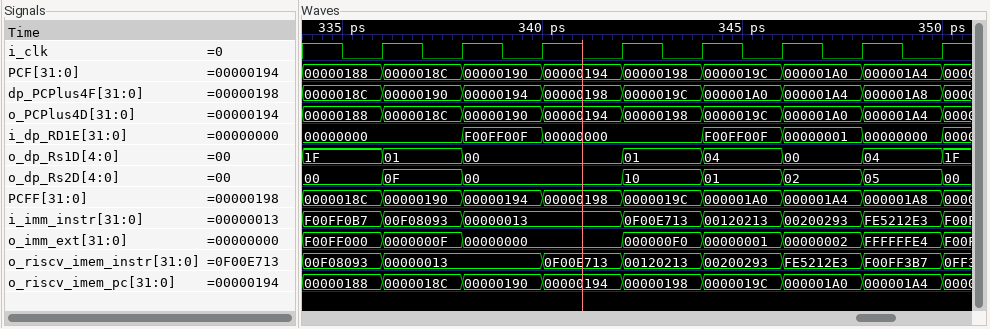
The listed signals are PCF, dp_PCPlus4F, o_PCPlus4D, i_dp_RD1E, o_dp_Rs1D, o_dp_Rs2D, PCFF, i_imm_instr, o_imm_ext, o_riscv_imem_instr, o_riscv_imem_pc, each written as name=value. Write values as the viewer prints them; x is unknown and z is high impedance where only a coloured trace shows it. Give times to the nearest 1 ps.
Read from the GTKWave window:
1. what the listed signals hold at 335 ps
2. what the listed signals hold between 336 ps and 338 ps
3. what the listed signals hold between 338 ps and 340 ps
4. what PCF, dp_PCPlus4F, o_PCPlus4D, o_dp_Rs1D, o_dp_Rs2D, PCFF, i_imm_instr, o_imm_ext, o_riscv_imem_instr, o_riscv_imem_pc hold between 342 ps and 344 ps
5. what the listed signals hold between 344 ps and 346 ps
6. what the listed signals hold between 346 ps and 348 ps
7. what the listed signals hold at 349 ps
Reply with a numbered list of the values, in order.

1. PCF=00000188, dp_PCPlus4F=0000018C, o_PCPlus4D=00000188, i_dp_RD1E=00000000, o_dp_Rs1D=1F, o_dp_Rs2D=00, PCFF=0000018C, i_imm_instr=F00FF0B7, o_imm_ext=F00FF000, o_riscv_imem_instr=00F08093, o_riscv_imem_pc=00000188
2. PCF=0000018C, dp_PCPlus4F=00000190, o_PCPlus4D=0000018C, i_dp_RD1E=00000000, o_dp_Rs1D=01, o_dp_Rs2D=0F, PCFF=00000190, i_imm_instr=00F08093, o_imm_ext=0000000F, o_riscv_imem_instr=00000013, o_riscv_imem_pc=0000018C
3. PCF=00000190, dp_PCPlus4F=00000194, o_PCPlus4D=00000190, i_dp_RD1E=F00FF00F, o_dp_Rs1D=00, o_dp_Rs2D=00, PCFF=00000194, i_imm_instr=00000013, o_imm_ext=00000000, o_riscv_imem_instr=00000013, o_riscv_imem_pc=00000190
4. PCF=00000198, dp_PCPlus4F=0000019C, o_PCPlus4D=00000198, o_dp_Rs1D=01, o_dp_Rs2D=10, PCFF=0000019C, i_imm_instr=0F00E713, o_imm_ext=000000F0, o_riscv_imem_instr=00120213, o_riscv_imem_pc=00000198
5. PCF=0000019C, dp_PCPlus4F=000001A0, o_PCPlus4D=0000019C, i_dp_RD1E=F00FF00F, o_dp_Rs1D=04, o_dp_Rs2D=01, PCFF=000001A0, i_imm_instr=00120213, o_imm_ext=00000001, o_riscv_imem_instr=00200293, o_riscv_imem_pc=0000019C
6. PCF=000001A0, dp_PCPlus4F=000001A4, o_PCPlus4D=000001A0, i_dp_RD1E=00000001, o_dp_Rs1D=00, o_dp_Rs2D=02, PCFF=000001A4, i_imm_instr=00200293, o_imm_ext=00000002, o_riscv_imem_instr=FE5212E3, o_riscv_imem_pc=000001A0
7. PCF=000001A4, dp_PCPlus4F=000001A8, o_PCPlus4D=000001A4, i_dp_RD1E=00000000, o_dp_Rs1D=04, o_dp_Rs2D=05, PCFF=000001A8, i_imm_instr=FE5212E3, o_imm_ext=FFFFFFE4, o_riscv_imem_instr=F00FF3B7, o_riscv_imem_pc=000001A4
